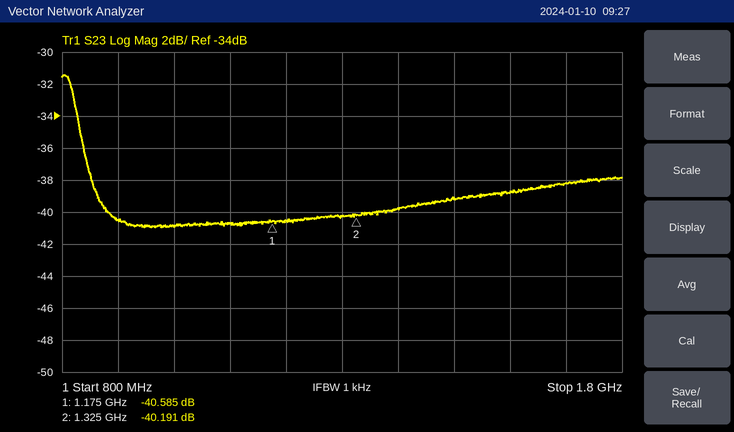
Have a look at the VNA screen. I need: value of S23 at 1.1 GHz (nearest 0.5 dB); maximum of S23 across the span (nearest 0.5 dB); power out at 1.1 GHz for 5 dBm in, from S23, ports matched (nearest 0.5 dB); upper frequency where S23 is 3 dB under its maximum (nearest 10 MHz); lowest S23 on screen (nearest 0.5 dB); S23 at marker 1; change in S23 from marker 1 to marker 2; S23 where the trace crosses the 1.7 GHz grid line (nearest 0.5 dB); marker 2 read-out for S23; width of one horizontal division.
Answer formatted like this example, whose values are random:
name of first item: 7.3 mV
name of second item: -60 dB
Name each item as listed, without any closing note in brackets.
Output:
value of S23 at 1.1 GHz: -40.5 dB
maximum of S23 across the span: -31.5 dB
power out at 1.1 GHz for 5 dBm in, from S23, ports matched: -35.5 dBm
upper frequency where S23 is 3 dB under its maximum: 830 MHz
lowest S23 on screen: -41.0 dB
S23 at marker 1: -40.585 dB
change in S23 from marker 1 to marker 2: 0.394 dB
S23 where the trace crosses the 1.7 GHz grid line: -38.0 dB
marker 2 read-out for S23: -40.191 dB
width of one horizontal division: 100 MHz
